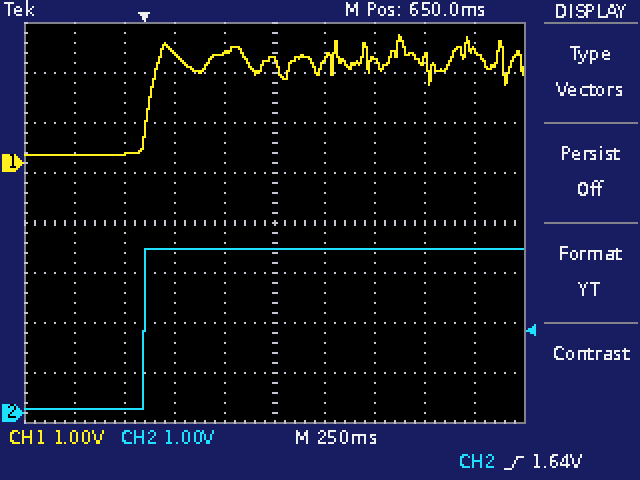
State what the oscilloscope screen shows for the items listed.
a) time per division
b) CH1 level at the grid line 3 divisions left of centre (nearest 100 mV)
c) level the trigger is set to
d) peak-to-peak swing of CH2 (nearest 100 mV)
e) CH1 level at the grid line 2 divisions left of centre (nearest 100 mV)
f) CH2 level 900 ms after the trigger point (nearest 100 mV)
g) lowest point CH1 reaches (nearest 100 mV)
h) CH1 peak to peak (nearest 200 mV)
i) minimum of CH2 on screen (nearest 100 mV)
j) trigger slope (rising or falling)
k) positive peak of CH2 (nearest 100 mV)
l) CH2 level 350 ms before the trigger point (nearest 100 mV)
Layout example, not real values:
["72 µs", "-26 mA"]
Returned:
["250 ms", "200 mV", "1.64 V", "3.2 V", "2.2 V", "3.3 V", "200 mV", "2.4 V", "100 mV", "rising", "3.3 V", "100 mV"]
